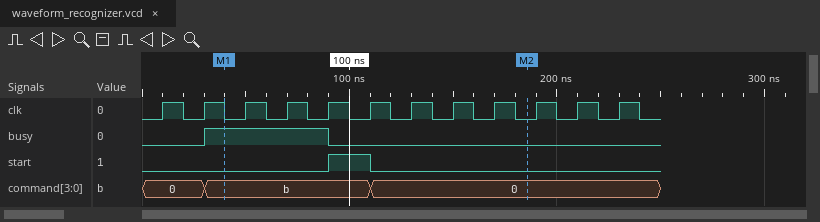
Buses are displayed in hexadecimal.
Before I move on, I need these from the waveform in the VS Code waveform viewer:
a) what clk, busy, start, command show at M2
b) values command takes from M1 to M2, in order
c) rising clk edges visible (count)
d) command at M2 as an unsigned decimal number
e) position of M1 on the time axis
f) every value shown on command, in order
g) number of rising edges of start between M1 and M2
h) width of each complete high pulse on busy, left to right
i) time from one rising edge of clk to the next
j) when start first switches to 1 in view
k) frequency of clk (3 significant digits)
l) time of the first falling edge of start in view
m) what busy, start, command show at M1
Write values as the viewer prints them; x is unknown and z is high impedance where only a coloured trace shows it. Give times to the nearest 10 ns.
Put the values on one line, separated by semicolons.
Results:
clk=0, busy=0, start=0, command=0; b, 0; 12; 0; 40 ns; 0, b, 0; 1; 60 ns; 20 ns; 90 ns; 50.0 MHz; 110 ns; busy=1, start=0, command=b
